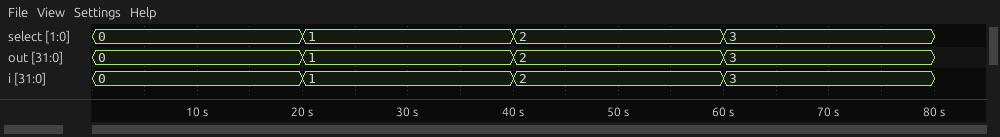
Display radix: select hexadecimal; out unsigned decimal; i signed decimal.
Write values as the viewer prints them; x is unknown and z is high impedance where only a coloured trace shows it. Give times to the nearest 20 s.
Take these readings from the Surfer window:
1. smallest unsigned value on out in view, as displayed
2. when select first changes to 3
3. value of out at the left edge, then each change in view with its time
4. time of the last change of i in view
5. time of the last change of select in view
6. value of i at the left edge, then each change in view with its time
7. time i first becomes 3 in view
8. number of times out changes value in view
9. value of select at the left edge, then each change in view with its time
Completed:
0
60 s
0, 1 at 20 s, 2 at 40 s, 3 at 60 s
60 s
60 s
0, 1 at 20 s, 2 at 40 s, 3 at 60 s
60 s
3
0, 1 at 20 s, 2 at 40 s, 3 at 60 s
